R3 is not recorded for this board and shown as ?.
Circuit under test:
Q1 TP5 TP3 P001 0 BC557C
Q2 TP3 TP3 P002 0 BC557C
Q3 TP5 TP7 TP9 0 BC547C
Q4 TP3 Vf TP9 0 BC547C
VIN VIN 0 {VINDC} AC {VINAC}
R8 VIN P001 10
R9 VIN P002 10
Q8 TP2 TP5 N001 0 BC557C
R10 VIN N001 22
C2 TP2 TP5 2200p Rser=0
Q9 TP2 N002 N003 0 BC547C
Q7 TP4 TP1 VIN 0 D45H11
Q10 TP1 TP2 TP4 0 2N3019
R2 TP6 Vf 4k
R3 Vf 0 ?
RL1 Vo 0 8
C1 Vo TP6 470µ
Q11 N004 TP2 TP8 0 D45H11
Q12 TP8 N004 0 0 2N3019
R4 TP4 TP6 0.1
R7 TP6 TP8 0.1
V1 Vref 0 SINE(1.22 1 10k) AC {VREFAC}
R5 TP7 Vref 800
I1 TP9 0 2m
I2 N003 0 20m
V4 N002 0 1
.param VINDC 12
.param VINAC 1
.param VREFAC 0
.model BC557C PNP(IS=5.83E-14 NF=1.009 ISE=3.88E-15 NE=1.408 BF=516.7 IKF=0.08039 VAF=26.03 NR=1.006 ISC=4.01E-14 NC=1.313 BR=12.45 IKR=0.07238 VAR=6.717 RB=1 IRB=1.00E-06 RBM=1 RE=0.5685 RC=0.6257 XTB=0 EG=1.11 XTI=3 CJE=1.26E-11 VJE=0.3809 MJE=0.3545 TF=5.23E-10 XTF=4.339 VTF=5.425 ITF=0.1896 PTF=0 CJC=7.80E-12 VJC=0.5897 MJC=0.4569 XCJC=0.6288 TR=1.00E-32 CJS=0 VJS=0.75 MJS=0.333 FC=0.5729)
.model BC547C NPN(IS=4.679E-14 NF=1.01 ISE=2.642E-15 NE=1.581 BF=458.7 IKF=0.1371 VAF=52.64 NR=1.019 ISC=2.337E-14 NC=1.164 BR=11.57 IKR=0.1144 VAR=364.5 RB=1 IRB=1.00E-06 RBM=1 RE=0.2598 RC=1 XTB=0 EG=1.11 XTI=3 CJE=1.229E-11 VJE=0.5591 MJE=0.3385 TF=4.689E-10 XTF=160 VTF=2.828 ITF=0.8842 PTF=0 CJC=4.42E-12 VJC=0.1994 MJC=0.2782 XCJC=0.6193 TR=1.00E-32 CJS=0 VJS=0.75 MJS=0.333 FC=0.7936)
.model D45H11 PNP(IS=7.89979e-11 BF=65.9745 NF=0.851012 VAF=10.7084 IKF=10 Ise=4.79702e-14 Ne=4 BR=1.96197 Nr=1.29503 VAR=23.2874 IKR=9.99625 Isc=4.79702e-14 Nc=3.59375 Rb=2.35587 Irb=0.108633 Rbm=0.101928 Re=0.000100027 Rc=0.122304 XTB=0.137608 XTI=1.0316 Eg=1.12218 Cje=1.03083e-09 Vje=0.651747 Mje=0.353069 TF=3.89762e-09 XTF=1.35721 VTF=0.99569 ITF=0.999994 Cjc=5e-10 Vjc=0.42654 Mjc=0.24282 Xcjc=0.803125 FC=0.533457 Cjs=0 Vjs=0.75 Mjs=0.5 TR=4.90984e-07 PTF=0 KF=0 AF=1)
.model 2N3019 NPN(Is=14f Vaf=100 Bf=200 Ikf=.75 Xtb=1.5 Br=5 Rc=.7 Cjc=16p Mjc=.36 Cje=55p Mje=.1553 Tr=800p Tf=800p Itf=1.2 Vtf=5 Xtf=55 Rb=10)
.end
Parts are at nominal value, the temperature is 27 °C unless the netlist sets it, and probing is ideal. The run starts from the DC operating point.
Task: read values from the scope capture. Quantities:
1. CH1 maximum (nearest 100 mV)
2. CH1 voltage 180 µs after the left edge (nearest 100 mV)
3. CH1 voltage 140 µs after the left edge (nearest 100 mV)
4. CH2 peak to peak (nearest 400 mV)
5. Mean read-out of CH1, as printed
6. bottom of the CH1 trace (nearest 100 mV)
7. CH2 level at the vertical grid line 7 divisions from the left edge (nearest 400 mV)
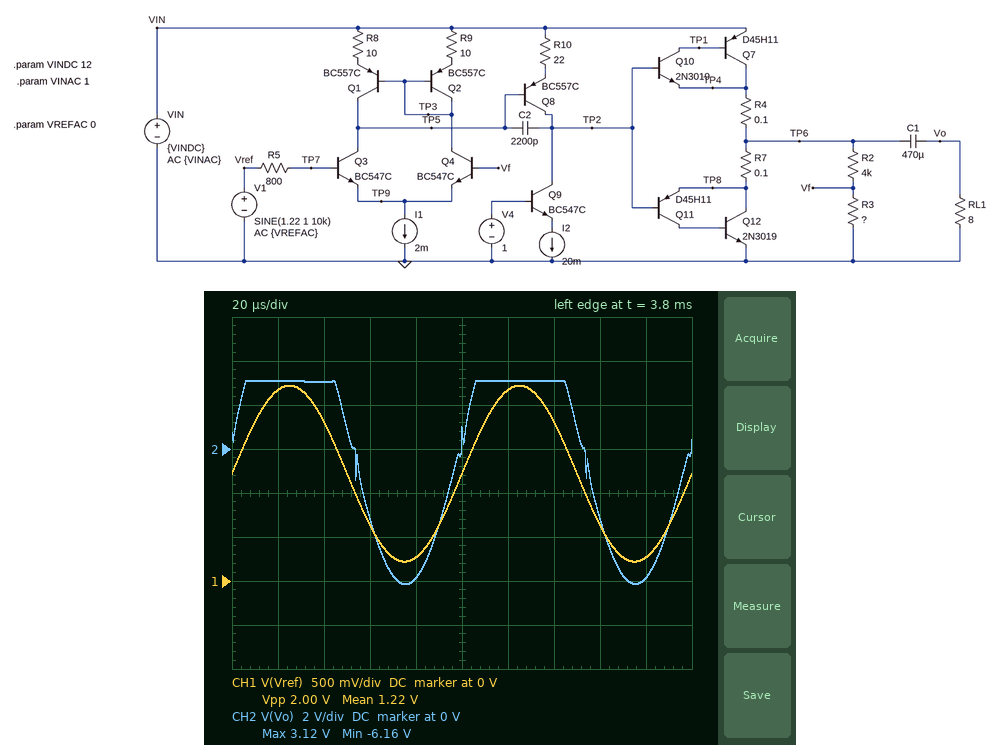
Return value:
2.2 V
300 mV
1.8 V
9.2 V
1.22 V
200 mV
3.2 V
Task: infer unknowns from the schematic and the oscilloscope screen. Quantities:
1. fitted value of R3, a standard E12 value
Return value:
680 Ω
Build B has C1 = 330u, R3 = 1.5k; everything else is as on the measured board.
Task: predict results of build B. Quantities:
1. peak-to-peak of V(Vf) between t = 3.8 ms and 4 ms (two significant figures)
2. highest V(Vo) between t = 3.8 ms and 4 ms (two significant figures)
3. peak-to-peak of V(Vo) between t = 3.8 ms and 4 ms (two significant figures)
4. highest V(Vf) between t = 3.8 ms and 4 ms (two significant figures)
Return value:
2.0 V
3.7 V
7.3 V
2.2 V
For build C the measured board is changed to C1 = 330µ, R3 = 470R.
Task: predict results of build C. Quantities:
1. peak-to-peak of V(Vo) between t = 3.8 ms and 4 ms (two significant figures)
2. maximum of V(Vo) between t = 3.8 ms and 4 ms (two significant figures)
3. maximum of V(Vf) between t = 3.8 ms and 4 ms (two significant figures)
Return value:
8.7 V
2.0 V
1.1 V
